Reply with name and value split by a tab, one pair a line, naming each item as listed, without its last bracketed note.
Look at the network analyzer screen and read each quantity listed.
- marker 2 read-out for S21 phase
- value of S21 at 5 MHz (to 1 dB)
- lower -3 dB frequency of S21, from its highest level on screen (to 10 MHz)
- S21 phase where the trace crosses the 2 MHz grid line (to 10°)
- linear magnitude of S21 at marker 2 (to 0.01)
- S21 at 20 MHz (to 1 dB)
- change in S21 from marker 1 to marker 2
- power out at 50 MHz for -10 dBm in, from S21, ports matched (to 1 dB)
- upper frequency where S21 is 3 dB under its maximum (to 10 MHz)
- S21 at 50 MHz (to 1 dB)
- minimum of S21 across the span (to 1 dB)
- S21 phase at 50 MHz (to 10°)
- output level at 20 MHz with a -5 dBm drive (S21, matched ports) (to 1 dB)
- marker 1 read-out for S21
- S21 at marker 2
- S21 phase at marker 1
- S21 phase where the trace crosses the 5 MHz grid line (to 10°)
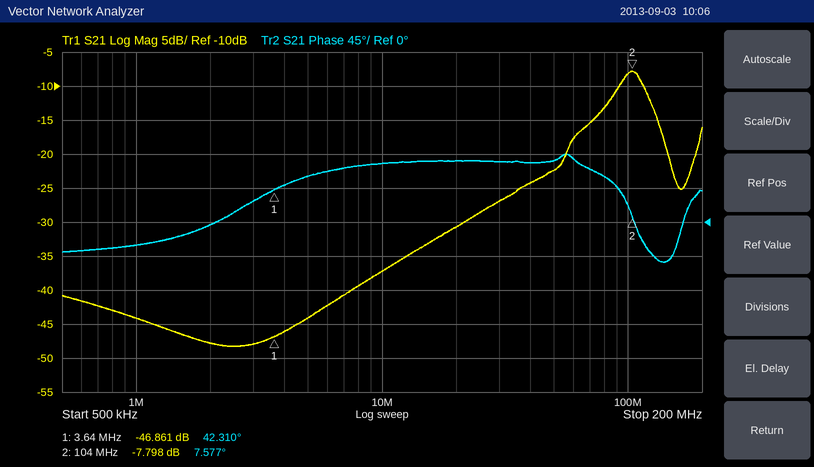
marker 2 read-out for S21 phase	7.577°
value of S21 at 5 MHz	-44 dB
lower -3 dB frequency of S21, from its highest level on screen	90 MHz
S21 phase where the trace crosses the 2 MHz grid line	0°
linear magnitude of S21 at marker 2	0.41
S21 at 20 MHz	-31 dB
change in S21 from marker 1 to marker 2	39.063 dB
power out at 50 MHz for -10 dBm in, from S21, ports matched	-32 dBm
upper frequency where S21 is 3 dB under its maximum	120 MHz
S21 at 50 MHz	-22 dB
minimum of S21 across the span	-48 dB
S21 phase at 50 MHz	80°
output level at 20 MHz with a -5 dBm drive (S21, matched ports)	-36 dBm
marker 1 read-out for S21	-46.861 dB
S21 at marker 2	-7.798 dB
S21 phase at marker 1	42.310°
S21 phase where the trace crosses the 5 MHz grid line	60°
